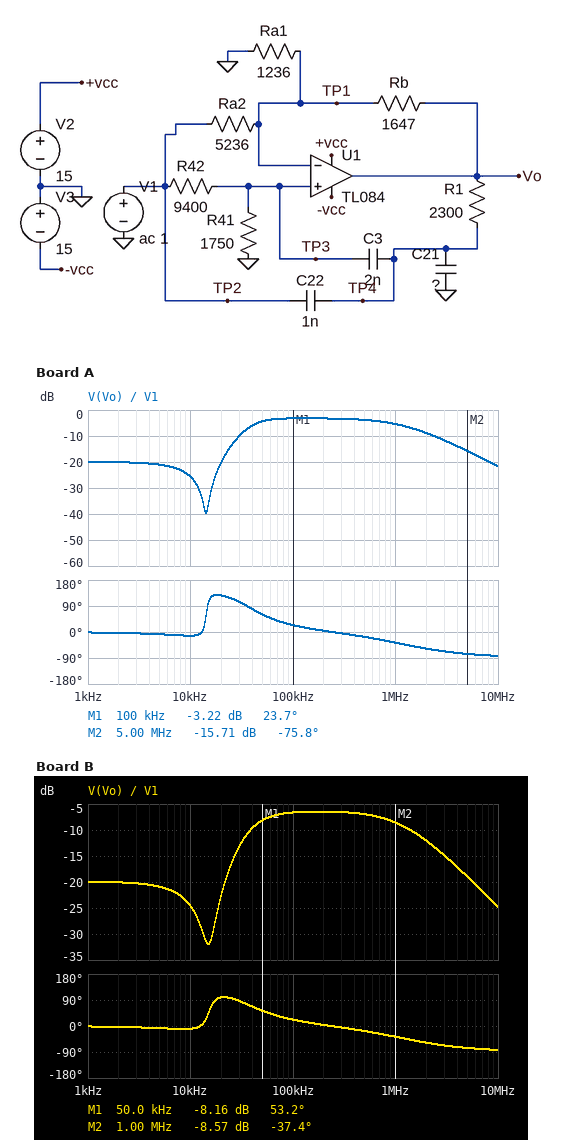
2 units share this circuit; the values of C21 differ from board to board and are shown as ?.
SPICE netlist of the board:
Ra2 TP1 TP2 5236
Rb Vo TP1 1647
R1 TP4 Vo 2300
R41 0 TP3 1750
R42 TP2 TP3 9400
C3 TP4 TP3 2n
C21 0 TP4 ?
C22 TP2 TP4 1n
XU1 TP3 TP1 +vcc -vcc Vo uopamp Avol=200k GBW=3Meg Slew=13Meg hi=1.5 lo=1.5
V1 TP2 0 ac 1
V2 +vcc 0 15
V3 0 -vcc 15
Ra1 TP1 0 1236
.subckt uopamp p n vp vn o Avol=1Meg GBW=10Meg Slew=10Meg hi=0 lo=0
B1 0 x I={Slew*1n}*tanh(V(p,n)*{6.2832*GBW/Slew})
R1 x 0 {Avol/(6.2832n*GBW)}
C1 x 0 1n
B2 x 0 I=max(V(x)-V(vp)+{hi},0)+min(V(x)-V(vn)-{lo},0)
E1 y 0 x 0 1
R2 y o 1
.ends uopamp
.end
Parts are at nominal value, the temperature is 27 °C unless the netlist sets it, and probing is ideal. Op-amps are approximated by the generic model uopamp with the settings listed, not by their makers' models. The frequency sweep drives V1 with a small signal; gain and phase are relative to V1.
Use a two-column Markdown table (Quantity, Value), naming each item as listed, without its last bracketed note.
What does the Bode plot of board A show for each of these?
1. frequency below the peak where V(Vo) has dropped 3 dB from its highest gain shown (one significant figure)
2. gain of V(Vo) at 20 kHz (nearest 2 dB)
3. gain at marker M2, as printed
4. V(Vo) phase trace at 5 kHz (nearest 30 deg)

| Quantity | Value |
|---|---|
| frequency below the peak where V(Vo) has dropped 3 dB from its highest gain shown | 40 kHz |
| gain of V(Vo) at 20 kHz | -20 dB |
| gain at marker M2, as printed | -15.71 dB |
| V(Vo) phase trace at 5 kHz | 0 deg |
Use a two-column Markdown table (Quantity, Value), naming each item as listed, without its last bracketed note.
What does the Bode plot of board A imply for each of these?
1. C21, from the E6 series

| Quantity | Value |
|---|---|
| C21, from the E6 series | 1.5 nF |
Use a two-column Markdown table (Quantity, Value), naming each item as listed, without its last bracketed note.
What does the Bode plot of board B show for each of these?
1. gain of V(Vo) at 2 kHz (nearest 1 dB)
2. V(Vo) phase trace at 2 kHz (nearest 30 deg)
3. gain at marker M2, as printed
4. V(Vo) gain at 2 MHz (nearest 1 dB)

| Quantity | Value |
|---|---|
| gain of V(Vo) at 2 kHz | -20 dB |
| V(Vo) phase trace at 2 kHz | 0 deg |
| gain at marker M2, as printed | -8.57 dB |
| V(Vo) gain at 2 MHz | -12 dB |
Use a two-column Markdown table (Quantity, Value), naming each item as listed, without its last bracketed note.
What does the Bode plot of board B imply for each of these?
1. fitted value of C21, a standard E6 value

| Quantity | Value |
|---|---|
| fitted value of C21, a standard E6 value | 2.2 nF |
